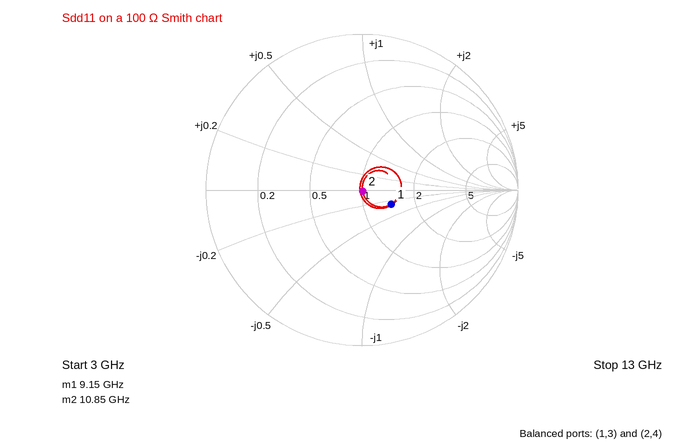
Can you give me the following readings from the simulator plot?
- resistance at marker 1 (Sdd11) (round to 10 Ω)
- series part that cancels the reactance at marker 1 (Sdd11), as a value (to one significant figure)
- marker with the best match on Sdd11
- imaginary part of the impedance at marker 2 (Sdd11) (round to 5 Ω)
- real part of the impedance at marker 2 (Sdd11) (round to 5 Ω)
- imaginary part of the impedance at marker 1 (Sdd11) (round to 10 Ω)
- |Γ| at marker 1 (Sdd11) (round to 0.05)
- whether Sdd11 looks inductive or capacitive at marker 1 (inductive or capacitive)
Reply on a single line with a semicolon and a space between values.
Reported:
140 Ω; 500 pH; marker 2; 0 Ω; 100 Ω; -30 Ω; 0.20; capacitive
